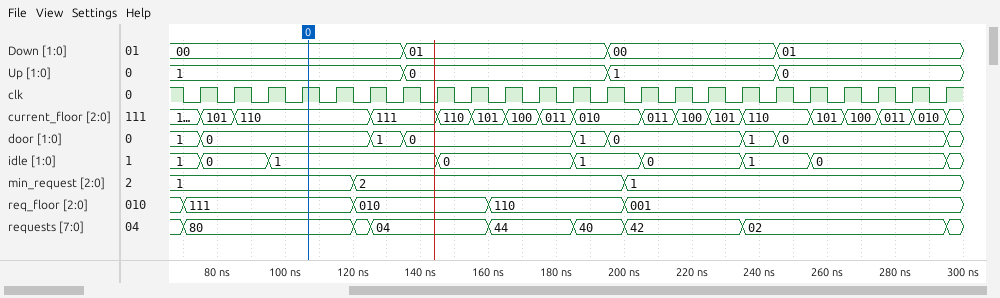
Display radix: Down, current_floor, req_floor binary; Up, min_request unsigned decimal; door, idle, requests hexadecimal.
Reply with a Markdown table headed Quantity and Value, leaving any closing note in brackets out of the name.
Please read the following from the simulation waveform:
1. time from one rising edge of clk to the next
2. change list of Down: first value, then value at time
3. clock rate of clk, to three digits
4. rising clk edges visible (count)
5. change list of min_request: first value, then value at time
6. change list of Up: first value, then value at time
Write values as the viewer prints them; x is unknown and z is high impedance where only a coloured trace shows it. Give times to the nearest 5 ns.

| Quantity | Value |
|---|---|
| time from one rising edge of clk to the next | 10 ns |
| change list of Down: first value, then value at time | 00, 01 at 135 ns, 00 at 195 ns, 01 at 245 ns |
| clock rate of clk, to three digits | 100 MHz |
| rising clk edges visible | 23 |
| change list of min_request: first value, then value at time | 1, 2 at 120 ns, 1 at 200 ns |
| change list of Up: first value, then value at time | 1, 0 at 135 ns, 1 at 195 ns, 0 at 245 ns |
